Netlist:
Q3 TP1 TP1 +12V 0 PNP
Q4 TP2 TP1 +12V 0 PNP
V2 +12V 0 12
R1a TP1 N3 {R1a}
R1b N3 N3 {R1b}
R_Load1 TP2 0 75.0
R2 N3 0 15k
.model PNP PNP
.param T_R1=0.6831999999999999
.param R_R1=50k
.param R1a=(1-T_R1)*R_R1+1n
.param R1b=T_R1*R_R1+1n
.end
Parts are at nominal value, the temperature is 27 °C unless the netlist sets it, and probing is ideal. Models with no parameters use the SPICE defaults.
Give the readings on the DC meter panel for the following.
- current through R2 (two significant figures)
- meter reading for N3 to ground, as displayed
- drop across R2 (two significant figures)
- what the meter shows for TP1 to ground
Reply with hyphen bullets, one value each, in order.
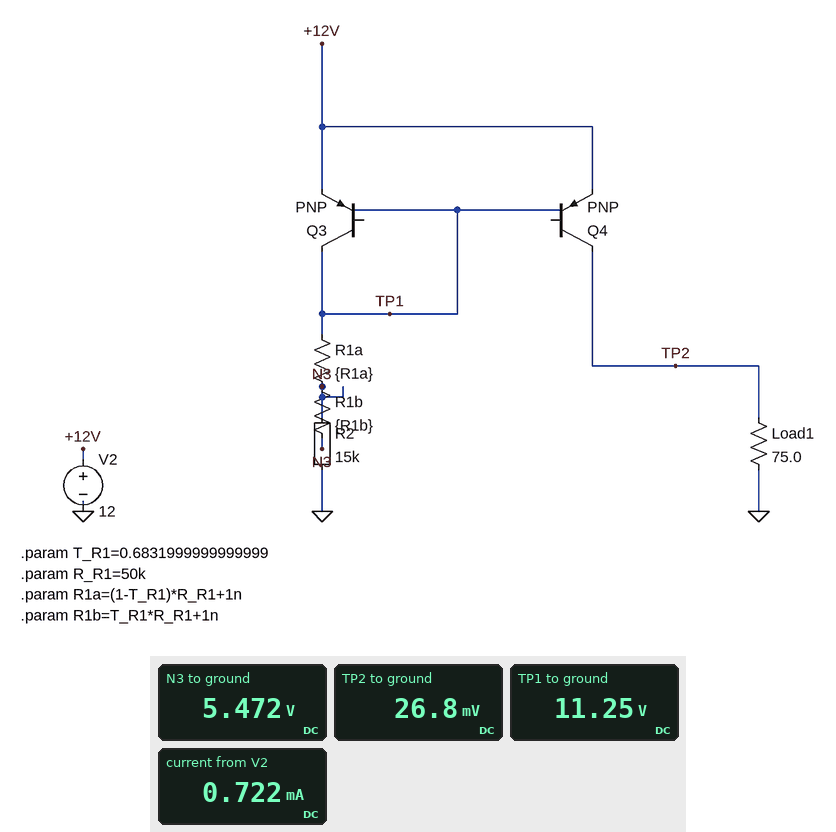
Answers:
- 360 µA
- 5.472 V
- 5.5 V
- 11.25 V
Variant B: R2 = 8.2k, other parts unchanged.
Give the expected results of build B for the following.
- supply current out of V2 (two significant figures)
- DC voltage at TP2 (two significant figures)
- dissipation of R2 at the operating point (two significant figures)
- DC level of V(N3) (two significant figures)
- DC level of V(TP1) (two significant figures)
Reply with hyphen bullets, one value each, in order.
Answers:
- 930 µA
- 34 mV
- 1.8 mW
- 3.8 V
- 11 V
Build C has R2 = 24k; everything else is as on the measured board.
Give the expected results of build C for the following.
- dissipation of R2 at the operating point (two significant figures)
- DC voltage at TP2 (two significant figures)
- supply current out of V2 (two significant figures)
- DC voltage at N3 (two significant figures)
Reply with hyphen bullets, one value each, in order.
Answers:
- 1.9 mW
- 21 mV
- 560 µA
- 6.8 V
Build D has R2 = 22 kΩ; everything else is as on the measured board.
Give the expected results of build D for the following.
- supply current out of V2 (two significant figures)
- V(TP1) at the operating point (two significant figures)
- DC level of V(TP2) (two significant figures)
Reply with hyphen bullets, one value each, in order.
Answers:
- 590 µA
- 11 V
- 22 mV
